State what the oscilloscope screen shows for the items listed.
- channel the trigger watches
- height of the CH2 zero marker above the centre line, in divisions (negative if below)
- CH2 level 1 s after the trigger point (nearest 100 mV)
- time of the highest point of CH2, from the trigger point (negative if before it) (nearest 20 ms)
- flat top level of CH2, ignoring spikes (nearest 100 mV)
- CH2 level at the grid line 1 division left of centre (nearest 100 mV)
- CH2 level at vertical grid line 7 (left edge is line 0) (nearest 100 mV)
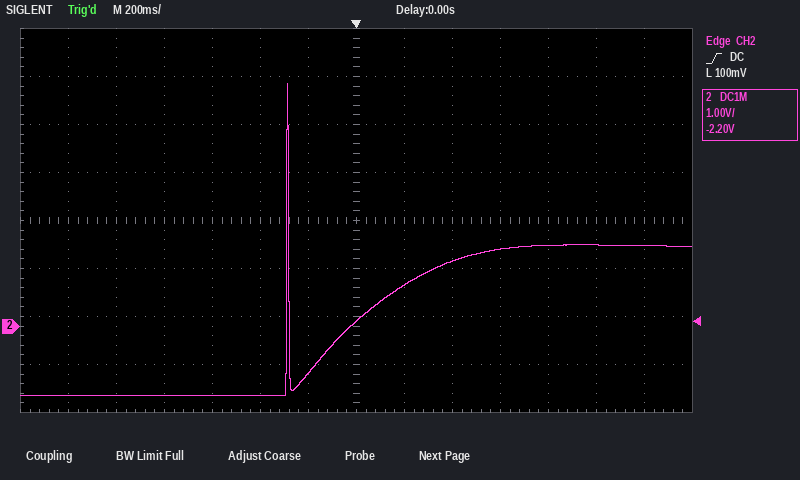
CH2
-2.2 div
1.7 V
-280 ms
1.7 V
-1.0 V
100 mV
